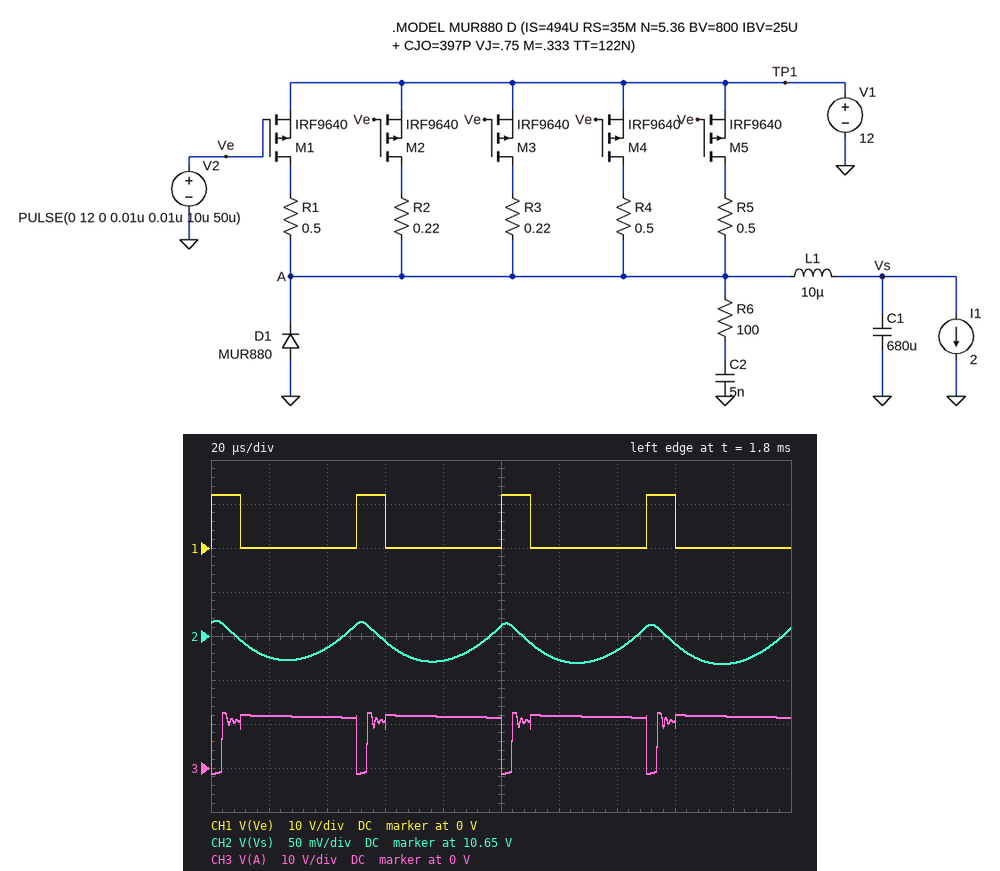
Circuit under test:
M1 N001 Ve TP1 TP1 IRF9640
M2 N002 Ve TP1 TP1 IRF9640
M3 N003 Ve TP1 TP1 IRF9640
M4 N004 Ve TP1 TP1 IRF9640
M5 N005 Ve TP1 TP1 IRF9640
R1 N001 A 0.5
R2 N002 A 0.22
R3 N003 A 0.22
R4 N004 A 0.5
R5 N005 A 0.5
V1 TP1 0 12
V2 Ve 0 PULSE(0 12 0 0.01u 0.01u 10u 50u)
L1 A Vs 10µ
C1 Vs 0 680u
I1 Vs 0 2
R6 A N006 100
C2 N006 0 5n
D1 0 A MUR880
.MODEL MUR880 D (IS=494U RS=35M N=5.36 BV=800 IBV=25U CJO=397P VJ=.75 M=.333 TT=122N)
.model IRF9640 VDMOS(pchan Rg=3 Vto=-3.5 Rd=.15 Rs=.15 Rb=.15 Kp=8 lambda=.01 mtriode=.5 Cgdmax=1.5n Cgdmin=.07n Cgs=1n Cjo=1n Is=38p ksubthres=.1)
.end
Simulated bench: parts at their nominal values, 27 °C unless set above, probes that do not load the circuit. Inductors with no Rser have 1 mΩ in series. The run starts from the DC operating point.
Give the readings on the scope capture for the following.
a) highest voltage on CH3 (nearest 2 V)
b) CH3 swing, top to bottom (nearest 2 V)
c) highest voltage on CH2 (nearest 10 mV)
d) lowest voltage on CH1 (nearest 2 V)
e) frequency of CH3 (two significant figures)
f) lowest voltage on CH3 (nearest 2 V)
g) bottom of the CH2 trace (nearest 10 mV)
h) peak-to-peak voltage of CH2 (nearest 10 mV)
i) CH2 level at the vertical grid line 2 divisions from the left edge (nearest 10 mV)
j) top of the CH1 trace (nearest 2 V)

12 V
14 V
10.67 V
0 V
20 kHz
-2 V
10.62 V
50 mV
10.64 V
12 V
